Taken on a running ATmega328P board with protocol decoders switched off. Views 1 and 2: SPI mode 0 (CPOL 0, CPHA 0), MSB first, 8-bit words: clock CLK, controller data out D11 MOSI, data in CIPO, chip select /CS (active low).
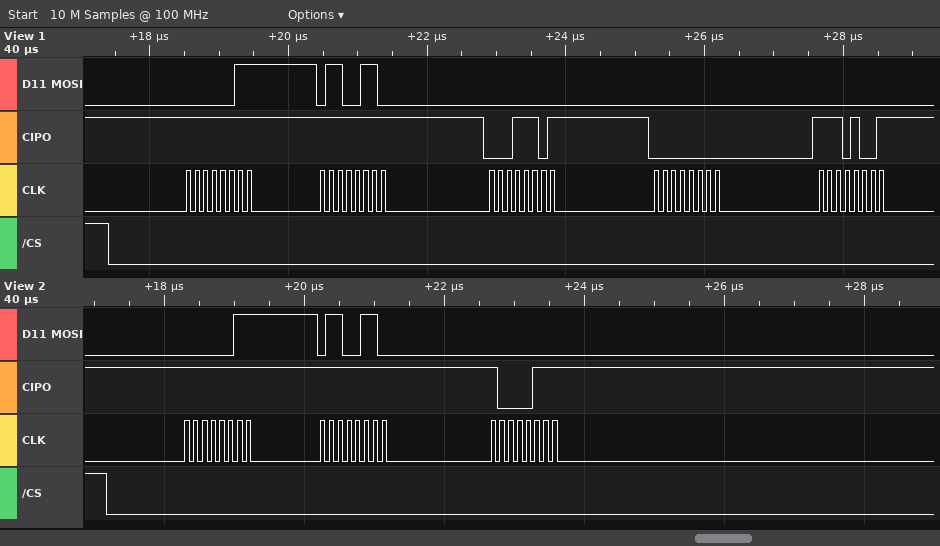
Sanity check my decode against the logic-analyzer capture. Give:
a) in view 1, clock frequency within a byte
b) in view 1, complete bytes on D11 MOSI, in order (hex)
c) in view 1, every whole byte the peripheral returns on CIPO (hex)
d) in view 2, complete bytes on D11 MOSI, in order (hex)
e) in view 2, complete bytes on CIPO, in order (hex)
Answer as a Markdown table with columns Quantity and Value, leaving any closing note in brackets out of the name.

| Quantity | Value |
|---|---|
| in view 1, clock frequency within a byte | 8 MHz |
| in view 1, complete bytes on D11 MOSI, in order | 0x03 0x66 0x00 0x00 0x00 |
| in view 1, every whole byte the peripheral returns on CIPO | 0xFF 0xFF 0x1D 0x00 0xE9 |
| in view 2, complete bytes on D11 MOSI, in order | 03 66 00 |
| in view 2, complete bytes on CIPO, in order | FF FF 87 |
